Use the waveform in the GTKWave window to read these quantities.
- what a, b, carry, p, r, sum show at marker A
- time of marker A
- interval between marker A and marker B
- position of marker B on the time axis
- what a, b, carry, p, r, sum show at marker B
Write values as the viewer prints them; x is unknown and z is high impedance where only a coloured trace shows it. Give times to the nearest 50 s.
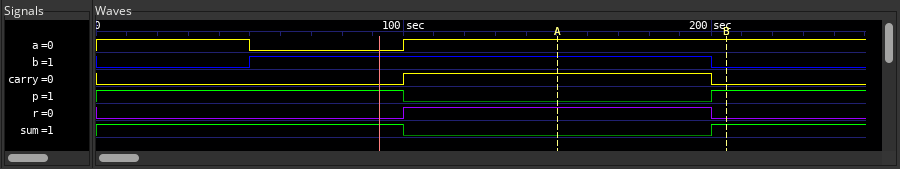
a=1, b=1, carry=1, p=0, r=1, sum=0
150 s
50 s
200 s
a=1, b=0, carry=0, p=1, r=0, sum=1
